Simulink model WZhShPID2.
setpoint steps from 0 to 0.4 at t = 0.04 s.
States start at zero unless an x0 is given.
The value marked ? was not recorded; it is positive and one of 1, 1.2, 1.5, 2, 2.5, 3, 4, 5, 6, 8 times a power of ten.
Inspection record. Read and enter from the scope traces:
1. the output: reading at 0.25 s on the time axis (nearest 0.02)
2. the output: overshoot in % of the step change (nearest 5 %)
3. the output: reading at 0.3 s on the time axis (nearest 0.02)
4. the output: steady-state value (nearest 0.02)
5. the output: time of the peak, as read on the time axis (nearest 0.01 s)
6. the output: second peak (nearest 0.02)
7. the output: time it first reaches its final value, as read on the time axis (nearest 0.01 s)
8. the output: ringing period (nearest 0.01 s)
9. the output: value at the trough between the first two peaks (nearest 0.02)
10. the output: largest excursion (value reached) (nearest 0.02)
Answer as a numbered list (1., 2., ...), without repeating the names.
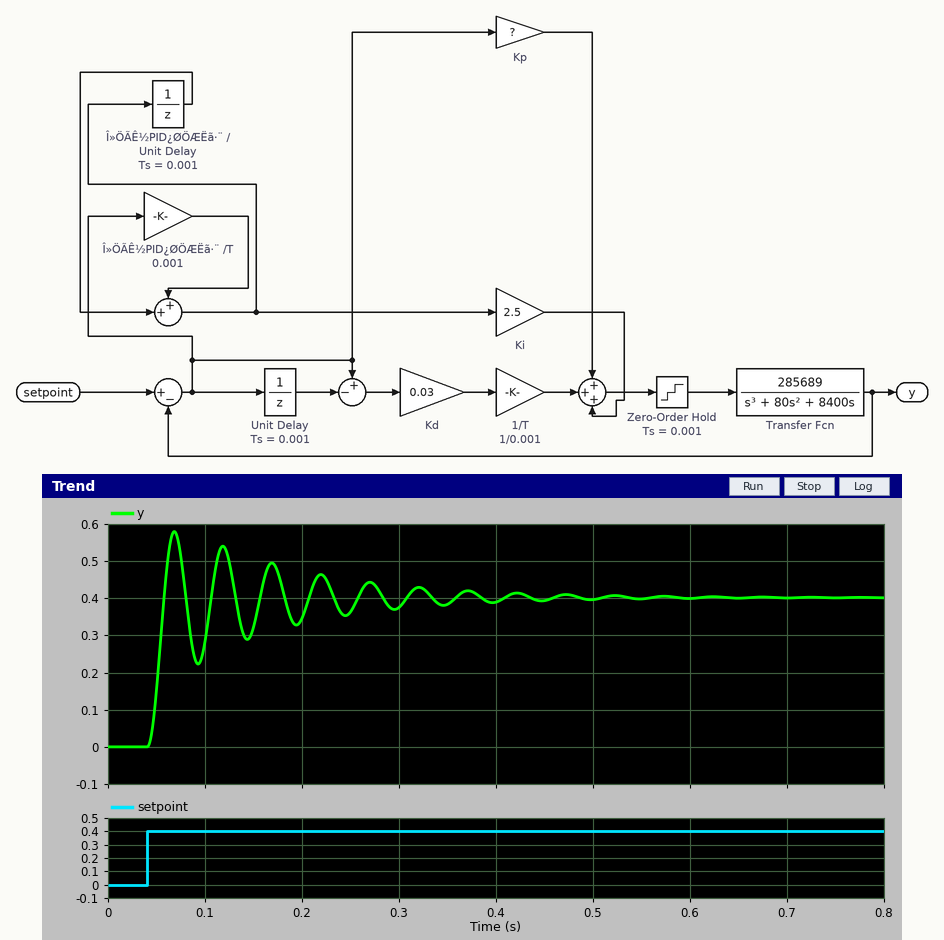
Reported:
1. 0.36
2. 45 %
3. 0.38
4. 0.40
5. 0.07 s
6. 0.54
7. 0.06 s
8. 0.05 s
9. 0.22
10. 0.58
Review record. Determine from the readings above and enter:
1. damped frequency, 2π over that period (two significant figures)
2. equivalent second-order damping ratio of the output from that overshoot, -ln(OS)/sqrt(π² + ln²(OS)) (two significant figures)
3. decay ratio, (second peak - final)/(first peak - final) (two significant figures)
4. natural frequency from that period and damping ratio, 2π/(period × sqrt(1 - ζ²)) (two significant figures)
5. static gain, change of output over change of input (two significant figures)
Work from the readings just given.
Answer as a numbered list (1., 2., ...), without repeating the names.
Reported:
1. 130 rad/s
2. 0.25
3. 0.78
4. 130 rad/s
5. 1.0
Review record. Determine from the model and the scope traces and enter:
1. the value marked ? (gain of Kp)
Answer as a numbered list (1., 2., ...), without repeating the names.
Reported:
1. 3
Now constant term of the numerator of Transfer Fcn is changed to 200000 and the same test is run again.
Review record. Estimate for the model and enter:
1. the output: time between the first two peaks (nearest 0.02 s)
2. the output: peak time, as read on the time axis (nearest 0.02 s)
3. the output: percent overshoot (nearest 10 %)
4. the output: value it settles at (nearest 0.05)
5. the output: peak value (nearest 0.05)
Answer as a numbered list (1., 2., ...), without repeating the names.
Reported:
1. 0.06 s
2. 0.08 s
3. 30 %
4. 0.40
5. 0.50
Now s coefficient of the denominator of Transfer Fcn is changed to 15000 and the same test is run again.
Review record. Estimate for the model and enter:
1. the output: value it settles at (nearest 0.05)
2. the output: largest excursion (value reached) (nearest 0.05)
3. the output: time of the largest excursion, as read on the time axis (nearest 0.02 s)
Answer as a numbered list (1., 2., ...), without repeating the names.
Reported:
1. 0.40
2. 0.45
3. 0.10 s
